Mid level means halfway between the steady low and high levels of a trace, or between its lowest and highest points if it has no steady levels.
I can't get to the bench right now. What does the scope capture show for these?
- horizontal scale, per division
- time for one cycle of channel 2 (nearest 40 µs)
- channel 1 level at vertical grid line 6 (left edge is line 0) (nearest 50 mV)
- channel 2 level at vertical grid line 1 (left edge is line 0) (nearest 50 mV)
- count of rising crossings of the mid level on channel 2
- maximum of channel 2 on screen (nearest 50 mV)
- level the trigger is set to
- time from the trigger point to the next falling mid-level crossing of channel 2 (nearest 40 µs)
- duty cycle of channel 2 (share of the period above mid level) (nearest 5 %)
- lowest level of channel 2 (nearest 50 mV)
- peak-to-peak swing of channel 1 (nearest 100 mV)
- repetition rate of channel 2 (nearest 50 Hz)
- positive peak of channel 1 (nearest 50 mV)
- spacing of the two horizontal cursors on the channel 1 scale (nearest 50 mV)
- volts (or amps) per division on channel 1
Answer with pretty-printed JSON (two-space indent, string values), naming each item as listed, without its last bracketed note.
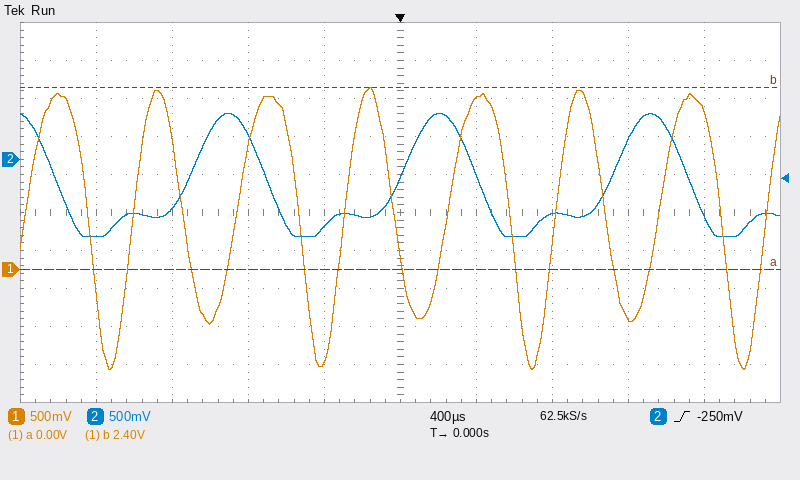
{
  "horizontal scale, per division": "400 µs",
  "time for one cycle of channel 2": "1.12 ms",
  "channel 1 level at vertical grid line 6 (left edge is line 0)": "2.25 V",
  "channel 2 level at vertical grid line 1 (left edge is line 0)": "-1.00 V",
  "count of rising crossings of the mid level on channel 2": "3",
  "maximum of channel 2 on screen": "600 mV",
  "level the trigger is set to": "-250 mV",
  "time from the trigger point to the next falling mid-level crossing of channel 2": "400 µs",
  "duty cycle of channel 2 (share of the period above mid level)": "35 %",
  "lowest level of channel 2": "-1.00 V",
  "peak-to-peak swing of channel 1": "3.70 V",
  "repetition rate of channel 2": "900 Hz",
  "positive peak of channel 1": "2.40 V",
  "spacing of the two horizontal cursors on the channel 1 scale": "2.40 V",
  "volts (or amps) per division on channel 1": "500 mV"
}
